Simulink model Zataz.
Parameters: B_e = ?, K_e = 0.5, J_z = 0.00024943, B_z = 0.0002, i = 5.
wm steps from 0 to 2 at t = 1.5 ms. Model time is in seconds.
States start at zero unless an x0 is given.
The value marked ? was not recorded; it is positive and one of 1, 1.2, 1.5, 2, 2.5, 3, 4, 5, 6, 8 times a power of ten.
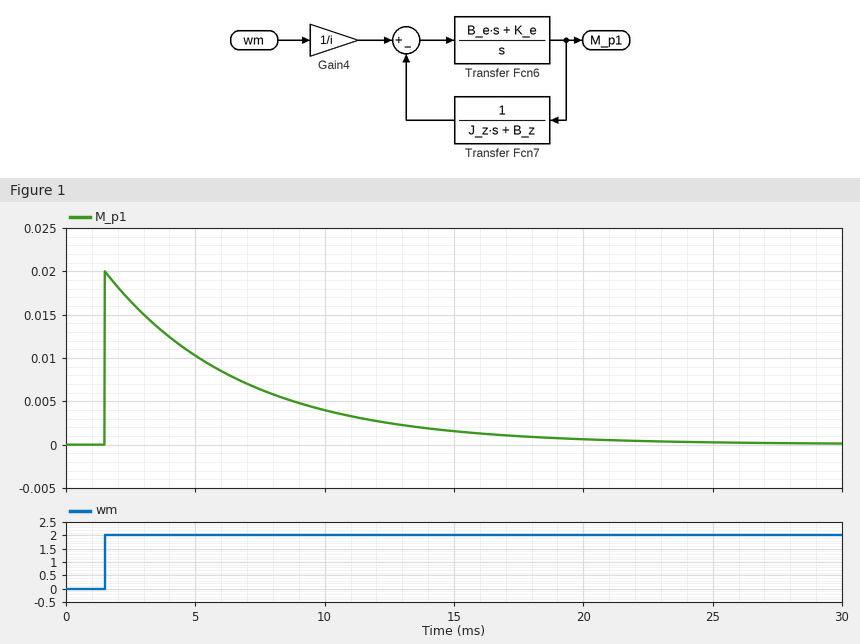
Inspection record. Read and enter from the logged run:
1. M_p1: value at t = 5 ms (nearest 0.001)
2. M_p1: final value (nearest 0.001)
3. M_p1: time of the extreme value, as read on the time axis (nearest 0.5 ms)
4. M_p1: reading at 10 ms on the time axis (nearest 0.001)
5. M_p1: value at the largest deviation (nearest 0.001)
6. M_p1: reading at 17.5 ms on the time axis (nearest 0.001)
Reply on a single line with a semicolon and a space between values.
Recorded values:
0.010; 0.000; 1.5 ms; 0.004; 0.020; 0.001
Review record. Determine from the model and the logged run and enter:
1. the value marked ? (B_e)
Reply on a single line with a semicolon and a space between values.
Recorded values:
0.05
